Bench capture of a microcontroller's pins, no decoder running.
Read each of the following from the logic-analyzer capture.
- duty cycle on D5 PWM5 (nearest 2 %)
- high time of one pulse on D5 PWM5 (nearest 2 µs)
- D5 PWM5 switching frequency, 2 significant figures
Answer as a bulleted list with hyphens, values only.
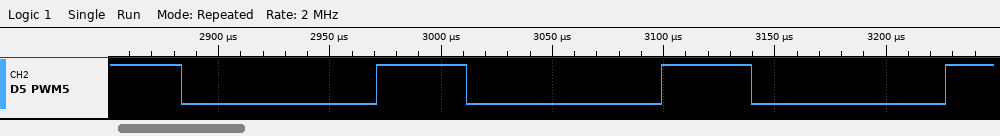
- 32 %
- 40 µs
- 7.8 kHz
